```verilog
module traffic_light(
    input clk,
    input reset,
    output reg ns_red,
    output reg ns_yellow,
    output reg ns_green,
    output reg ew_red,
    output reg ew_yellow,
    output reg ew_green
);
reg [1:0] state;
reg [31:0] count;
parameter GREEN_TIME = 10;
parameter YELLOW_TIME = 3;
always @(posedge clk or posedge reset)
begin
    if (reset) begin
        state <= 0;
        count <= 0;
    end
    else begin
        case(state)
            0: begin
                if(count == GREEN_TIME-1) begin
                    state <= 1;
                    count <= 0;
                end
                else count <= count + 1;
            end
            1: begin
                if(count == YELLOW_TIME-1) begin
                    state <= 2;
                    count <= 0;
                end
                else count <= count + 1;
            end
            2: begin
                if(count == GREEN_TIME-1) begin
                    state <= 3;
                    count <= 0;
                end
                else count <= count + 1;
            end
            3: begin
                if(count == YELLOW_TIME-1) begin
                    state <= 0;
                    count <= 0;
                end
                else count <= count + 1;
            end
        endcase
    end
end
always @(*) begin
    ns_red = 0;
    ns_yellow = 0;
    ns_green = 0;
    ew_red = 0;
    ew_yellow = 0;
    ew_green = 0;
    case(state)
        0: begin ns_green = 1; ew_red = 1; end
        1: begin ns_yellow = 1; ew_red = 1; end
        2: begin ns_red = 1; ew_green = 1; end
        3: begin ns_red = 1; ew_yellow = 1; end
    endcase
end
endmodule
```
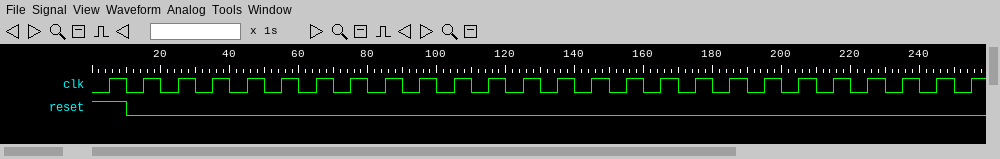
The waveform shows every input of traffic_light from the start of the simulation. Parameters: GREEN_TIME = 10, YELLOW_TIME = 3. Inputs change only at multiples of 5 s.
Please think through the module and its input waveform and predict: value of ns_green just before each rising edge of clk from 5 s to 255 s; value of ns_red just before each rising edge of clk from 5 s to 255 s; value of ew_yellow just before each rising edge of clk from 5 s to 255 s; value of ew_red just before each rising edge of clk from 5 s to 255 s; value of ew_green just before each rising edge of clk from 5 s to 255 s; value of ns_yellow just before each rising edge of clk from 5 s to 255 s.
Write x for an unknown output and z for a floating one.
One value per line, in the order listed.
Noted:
1 1 1 1 1 1 1 1 1 1 1 0 0 0 0 0 0 0 0 0 0 0 0 0 0 0
0 0 0 0 0 0 0 0 0 0 0 0 0 0 1 1 1 1 1 1 1 1 1 1 1 1
0 0 0 0 0 0 0 0 0 0 0 0 0 0 0 0 0 0 0 0 0 0 0 0 1 1
1 1 1 1 1 1 1 1 1 1 1 1 1 1 0 0 0 0 0 0 0 0 0 0 0 0
0 0 0 0 0 0 0 0 0 0 0 0 0 0 1 1 1 1 1 1 1 1 1 1 0 0
0 0 0 0 0 0 0 0 0 0 0 1 1 1 0 0 0 0 0 0 0 0 0 0 0 0
